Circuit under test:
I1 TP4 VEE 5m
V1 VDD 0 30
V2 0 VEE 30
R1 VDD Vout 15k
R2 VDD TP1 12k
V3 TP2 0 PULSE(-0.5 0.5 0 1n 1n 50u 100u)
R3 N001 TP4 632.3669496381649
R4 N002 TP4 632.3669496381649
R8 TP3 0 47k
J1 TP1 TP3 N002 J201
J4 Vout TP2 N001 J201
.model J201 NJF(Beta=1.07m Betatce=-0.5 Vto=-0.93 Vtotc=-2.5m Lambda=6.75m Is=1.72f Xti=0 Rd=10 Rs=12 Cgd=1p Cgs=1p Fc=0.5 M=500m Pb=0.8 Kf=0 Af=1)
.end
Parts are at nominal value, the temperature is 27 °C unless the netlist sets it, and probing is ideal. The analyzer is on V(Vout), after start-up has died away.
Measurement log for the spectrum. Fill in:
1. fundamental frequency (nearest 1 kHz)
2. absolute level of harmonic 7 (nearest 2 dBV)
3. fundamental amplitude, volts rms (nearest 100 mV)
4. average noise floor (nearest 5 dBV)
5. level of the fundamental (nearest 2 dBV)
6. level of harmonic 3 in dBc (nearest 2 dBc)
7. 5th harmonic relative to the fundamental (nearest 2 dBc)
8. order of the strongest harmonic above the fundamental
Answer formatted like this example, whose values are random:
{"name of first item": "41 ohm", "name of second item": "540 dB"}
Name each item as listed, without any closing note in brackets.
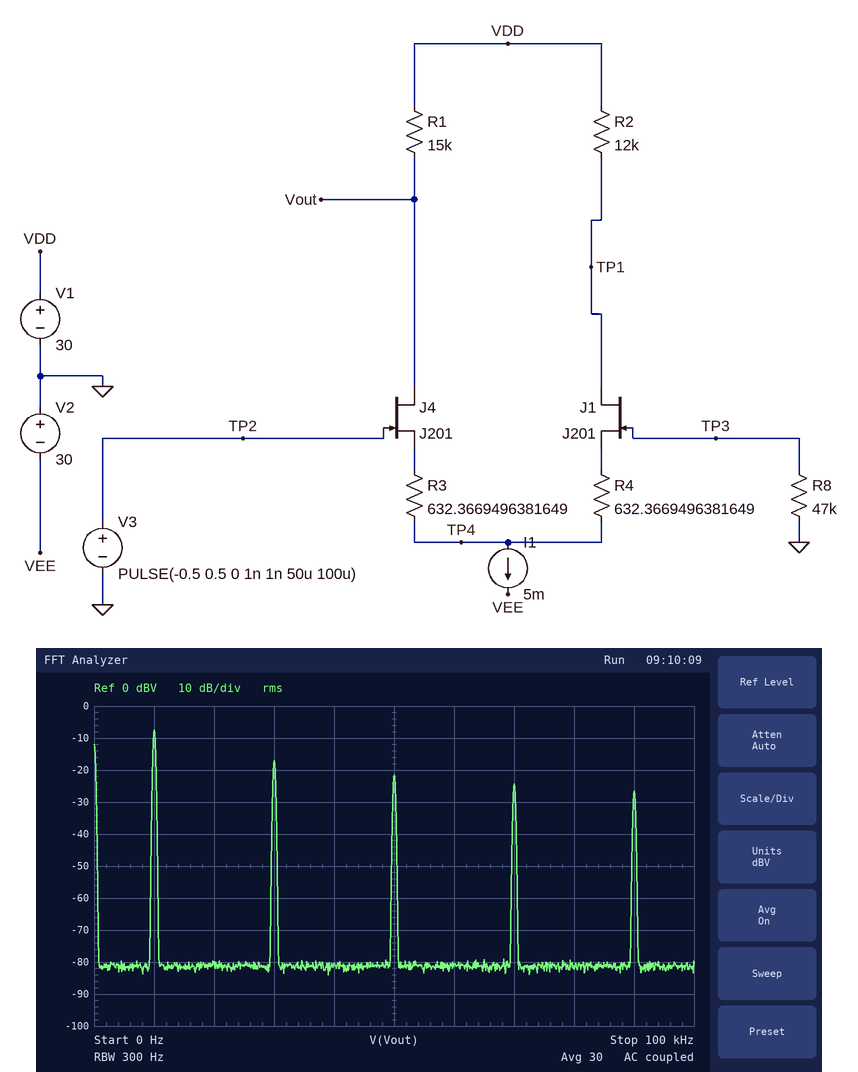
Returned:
{"fundamental frequency": "10 kHz", "absolute level of harmonic 7": "-24 dBV", "fundamental amplitude, volts rms": "400 mV", "average noise floor": "-80 dBV", "level of the fundamental": "-8 dBV", "level of harmonic 3 in dBc": "-10 dBc", "5th harmonic relative to the fundamental": "-14 dBc", "order of the strongest harmonic above the fundamental": "3"}
